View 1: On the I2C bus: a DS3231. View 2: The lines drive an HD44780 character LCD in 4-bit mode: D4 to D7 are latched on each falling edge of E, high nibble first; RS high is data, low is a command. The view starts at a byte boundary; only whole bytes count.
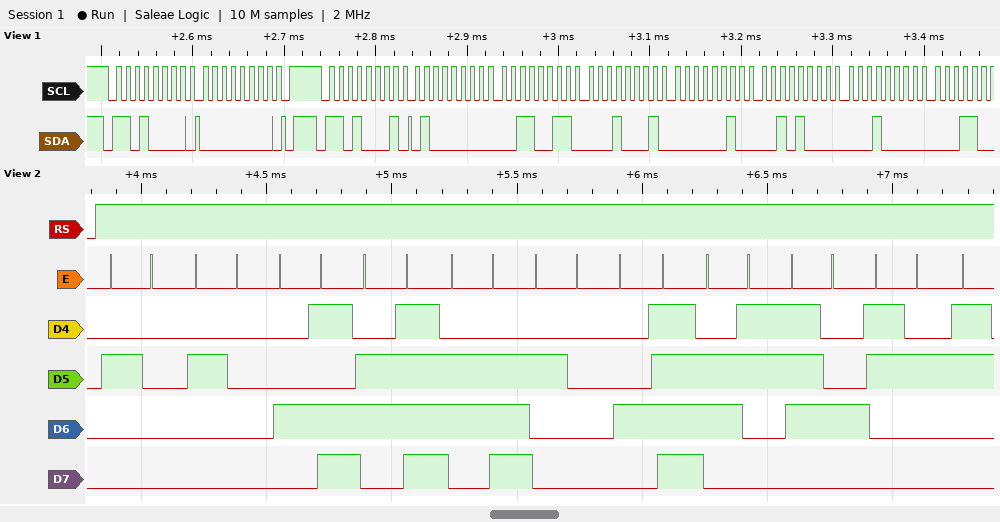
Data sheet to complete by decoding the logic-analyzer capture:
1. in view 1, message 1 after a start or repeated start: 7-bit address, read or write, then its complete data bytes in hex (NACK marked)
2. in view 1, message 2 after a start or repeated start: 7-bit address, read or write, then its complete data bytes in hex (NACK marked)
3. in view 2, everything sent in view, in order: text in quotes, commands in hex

0x68 write: 00
0x68 read: 40 33 11 02 28 10
"  Mon Oct2"
